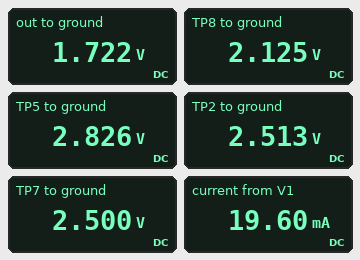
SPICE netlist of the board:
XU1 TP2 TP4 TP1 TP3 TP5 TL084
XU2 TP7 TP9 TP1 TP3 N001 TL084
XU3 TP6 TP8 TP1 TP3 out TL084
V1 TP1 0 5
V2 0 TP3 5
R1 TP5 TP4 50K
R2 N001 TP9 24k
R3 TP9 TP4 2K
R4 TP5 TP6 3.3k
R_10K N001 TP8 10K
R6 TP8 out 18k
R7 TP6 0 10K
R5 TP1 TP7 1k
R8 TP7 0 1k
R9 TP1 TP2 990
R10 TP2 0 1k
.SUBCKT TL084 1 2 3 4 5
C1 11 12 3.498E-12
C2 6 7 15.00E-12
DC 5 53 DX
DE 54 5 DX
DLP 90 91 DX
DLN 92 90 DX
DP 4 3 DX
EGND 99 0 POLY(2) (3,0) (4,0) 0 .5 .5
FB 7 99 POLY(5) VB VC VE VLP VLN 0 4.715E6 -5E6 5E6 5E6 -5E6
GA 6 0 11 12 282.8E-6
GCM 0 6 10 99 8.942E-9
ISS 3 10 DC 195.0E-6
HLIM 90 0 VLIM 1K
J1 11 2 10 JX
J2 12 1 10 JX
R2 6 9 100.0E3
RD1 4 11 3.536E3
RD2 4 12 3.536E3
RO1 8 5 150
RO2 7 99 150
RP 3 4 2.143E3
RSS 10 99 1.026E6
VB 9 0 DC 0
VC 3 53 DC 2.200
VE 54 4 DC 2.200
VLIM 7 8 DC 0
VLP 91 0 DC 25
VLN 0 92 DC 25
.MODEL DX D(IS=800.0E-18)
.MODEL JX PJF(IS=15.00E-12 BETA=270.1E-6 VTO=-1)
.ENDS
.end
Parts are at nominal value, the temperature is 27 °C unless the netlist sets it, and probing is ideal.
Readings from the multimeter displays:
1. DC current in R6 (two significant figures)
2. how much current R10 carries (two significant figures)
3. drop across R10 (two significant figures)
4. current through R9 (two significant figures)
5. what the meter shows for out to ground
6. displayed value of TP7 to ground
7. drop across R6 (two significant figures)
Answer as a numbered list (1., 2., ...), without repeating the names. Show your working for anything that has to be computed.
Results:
1. (2.125 V - 1.722 V) / 18 kΩ = 22 µA
2. (2.513 V) / 1 kΩ = 2.5 mA
3. 2.513 V = 2.5 V
4. (5 V - 2.513 V) / 990 Ω = 2.5 mA
5. 1.722 V
6. 2.500 V
7. 2.125 V - 1.722 V = 400 mV
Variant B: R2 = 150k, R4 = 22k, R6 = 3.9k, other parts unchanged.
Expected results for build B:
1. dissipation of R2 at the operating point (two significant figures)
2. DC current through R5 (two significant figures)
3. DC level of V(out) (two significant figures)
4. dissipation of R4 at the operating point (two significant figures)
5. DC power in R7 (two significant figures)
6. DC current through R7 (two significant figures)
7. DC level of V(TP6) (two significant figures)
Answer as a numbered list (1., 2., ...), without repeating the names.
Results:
1. 5.9 µW
2. 2.5 mA
3. 620 mV
4. 170 µW
5. 78 µW
6. 88 µA
7. 880 mV
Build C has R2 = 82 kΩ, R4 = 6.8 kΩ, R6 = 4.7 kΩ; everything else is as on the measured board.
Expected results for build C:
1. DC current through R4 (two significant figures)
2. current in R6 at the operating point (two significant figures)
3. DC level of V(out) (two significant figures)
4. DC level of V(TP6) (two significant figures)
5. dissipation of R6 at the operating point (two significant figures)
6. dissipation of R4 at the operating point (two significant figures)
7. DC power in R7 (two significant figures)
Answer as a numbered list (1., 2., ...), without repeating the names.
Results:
1. 170 µA
2. 30 µA
3. 1.5 V
4. 1.7 V
5. 4.3 µW
6. 190 µW
7. 280 µW
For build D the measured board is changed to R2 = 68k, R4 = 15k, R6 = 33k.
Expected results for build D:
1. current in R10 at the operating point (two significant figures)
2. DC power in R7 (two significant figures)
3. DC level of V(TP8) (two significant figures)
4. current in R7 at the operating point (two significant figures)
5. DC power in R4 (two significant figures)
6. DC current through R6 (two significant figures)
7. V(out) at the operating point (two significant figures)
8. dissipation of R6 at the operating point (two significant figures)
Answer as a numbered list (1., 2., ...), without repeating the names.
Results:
1. 2.5 mA
2. 130 µW
3. 1.1 V
4. 110 µA
5. 190 µW
6. 94 µA
7. -2.0 V
8. 290 µW
